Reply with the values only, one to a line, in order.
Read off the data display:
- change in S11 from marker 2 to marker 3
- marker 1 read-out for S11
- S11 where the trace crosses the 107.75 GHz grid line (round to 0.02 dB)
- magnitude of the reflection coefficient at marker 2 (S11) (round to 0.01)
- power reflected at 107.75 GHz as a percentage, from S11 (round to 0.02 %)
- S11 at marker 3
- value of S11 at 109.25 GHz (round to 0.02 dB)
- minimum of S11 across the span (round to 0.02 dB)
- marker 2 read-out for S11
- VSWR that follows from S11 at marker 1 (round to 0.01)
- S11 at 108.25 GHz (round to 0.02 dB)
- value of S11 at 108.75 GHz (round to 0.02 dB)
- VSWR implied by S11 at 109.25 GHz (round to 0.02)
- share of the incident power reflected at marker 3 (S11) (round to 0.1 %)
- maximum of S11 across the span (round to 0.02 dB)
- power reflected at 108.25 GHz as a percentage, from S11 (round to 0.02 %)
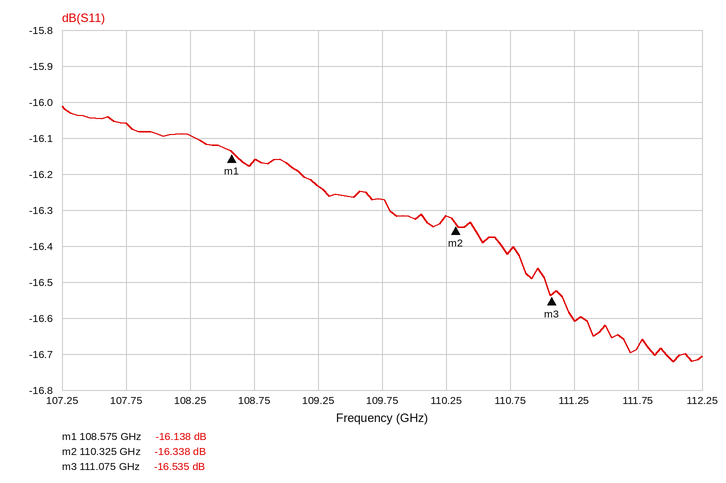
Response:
-0.197 dB
-16.138 dB
-16.06 dB
0.15
2.48 %
-16.535 dB
-16.24 dB
-16.72 dB
-16.338 dB
1.37
-16.10 dB
-16.16 dB
1.36
2.2 %
-16.02 dB
2.46 %
